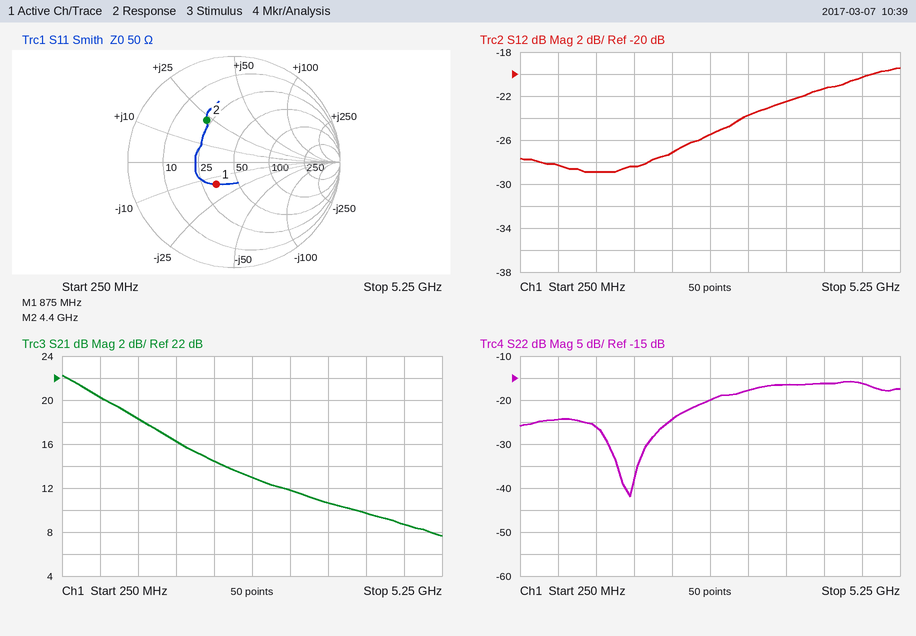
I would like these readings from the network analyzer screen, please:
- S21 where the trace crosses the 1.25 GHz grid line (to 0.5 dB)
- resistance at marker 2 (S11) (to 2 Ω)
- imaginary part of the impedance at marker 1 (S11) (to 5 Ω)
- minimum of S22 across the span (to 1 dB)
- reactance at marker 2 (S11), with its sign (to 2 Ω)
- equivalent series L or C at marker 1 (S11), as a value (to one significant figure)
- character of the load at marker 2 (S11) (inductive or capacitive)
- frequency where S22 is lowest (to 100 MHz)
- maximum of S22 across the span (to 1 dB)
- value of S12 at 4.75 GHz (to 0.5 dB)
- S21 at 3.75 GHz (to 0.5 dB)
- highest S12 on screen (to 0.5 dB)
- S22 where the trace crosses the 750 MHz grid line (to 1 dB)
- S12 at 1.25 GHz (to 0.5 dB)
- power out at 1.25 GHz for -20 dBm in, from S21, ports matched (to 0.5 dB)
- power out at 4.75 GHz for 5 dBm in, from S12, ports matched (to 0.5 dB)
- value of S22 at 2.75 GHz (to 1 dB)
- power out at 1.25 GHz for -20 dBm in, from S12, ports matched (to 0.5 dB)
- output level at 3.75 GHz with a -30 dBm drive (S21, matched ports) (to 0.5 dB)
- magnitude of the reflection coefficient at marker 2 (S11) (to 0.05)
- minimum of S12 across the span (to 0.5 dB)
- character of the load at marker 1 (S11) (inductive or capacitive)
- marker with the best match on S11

18.5 dB
22 Ω
-15 Ω
-42 dB
+22 Ω
10 pF
inductive
1.7 GHz
-16 dB
-20.5 dB
10.5 dB
-19.5 dB
-24 dB
-29.0 dB
-1.5 dBm
-15.5 dBm
-20 dB
-49.0 dBm
-19.5 dBm
0.45
-29.0 dB
capacitive
marker 1
